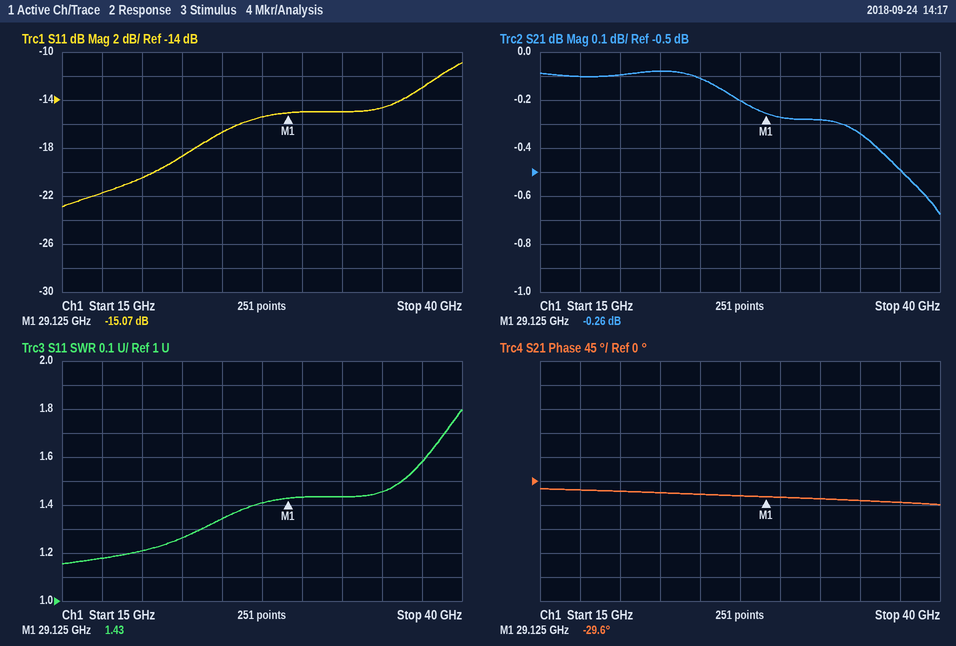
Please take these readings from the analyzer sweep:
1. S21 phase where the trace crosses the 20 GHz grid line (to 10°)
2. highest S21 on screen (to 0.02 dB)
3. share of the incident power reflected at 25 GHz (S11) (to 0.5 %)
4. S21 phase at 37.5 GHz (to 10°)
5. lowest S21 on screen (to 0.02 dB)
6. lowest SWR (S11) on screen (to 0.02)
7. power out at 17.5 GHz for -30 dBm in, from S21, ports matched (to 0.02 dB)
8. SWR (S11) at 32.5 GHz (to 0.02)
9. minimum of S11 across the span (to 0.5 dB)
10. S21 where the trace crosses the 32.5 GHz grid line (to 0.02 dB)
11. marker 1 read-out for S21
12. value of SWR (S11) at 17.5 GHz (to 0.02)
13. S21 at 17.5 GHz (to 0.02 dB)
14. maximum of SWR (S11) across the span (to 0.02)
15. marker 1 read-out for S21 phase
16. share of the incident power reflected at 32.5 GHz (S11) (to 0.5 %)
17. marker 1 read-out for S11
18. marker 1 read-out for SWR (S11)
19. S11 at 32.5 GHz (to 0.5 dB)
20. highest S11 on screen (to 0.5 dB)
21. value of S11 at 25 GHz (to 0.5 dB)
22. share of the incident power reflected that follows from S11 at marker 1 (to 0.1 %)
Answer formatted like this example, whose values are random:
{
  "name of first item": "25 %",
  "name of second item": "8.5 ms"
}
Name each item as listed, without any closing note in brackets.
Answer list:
{
  "S21 phase where the trace crosses the 20 GHz grid line": "-20°",
  "highest S21 on screen": "-0.08 dB",
  "share of the incident power reflected at 25 GHz (S11)": "2.0 %",
  "S21 phase at 37.5 GHz": "-40°",
  "lowest S21 on screen": "-0.68 dB",
  "lowest SWR (S11) on screen": "1.16",
  "power out at 17.5 GHz for -30 dBm in, from S21, ports matched": "-30.10 dBm",
  "SWR (S11) at 32.5 GHz": "1.44",
  "minimum of S11 across the span": "-23.0 dB",
  "S21 where the trace crosses the 32.5 GHz grid line": "-0.28 dB",
  "marker 1 read-out for S21": "-0.26 dB",
  "value of SWR (S11) at 17.5 GHz": "1.18",
  "S21 at 17.5 GHz": "-0.10 dB",
  "maximum of SWR (S11) across the span": "1.80",
  "marker 1 read-out for S21 phase": "-29.6°",
  "share of the incident power reflected at 32.5 GHz (S11)": "3.0 %",
  "marker 1 read-out for S11": "-15.07 dB",
  "marker 1 read-out for SWR": "1.43",
  "S11 at 32.5 GHz": "-15.0 dB",
  "highest S11 on screen": "-11.0 dB",
  "value of S11 at 25 GHz": "-16.5 dB",
  "share of the incident power reflected that follows from S11 at marker 1": "3.1 %"
}
